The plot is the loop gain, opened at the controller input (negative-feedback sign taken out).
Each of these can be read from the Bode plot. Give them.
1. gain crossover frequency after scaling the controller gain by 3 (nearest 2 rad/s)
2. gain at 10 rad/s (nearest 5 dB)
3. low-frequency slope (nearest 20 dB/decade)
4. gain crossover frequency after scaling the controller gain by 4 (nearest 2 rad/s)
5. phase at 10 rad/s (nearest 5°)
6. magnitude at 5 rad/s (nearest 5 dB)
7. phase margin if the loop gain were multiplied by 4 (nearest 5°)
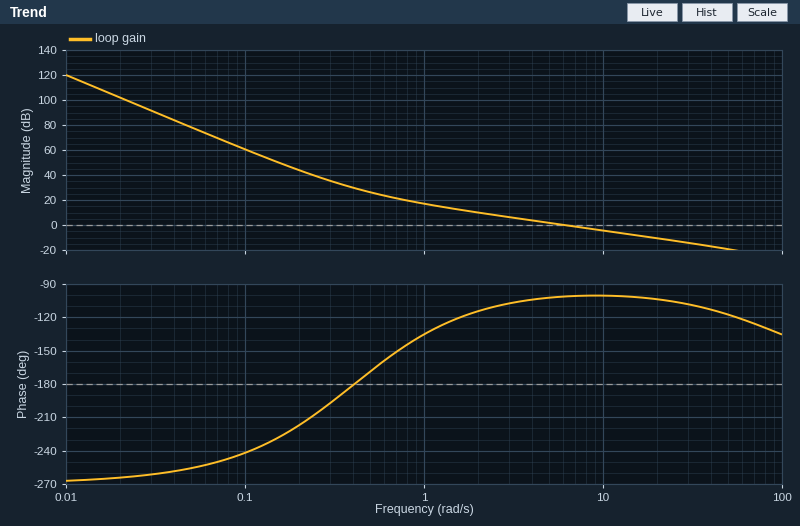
18 rad/s
-5 dB
-60 dB/decade
24 rad/s
-100°
0 dB
75°
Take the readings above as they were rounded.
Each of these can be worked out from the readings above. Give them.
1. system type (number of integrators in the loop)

3
